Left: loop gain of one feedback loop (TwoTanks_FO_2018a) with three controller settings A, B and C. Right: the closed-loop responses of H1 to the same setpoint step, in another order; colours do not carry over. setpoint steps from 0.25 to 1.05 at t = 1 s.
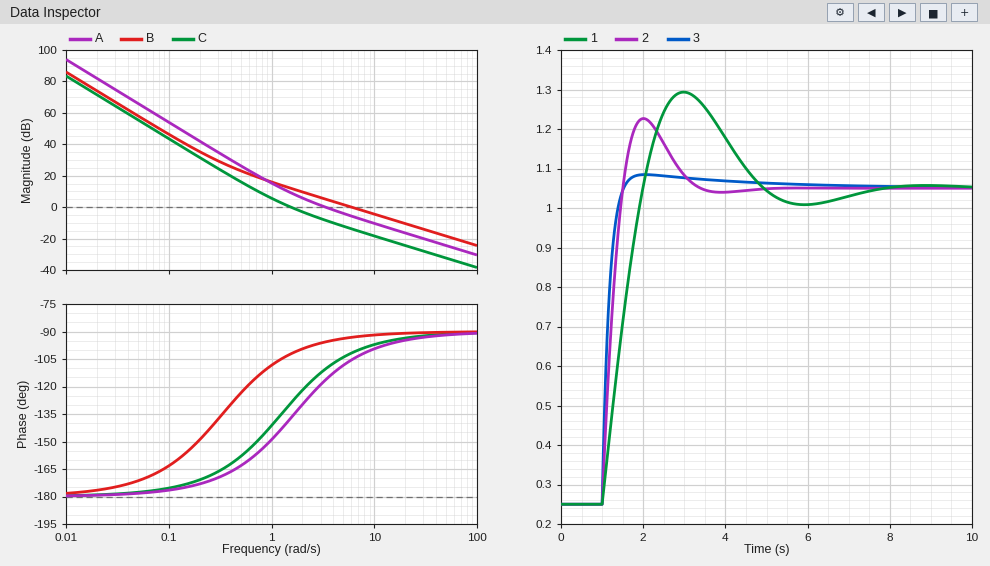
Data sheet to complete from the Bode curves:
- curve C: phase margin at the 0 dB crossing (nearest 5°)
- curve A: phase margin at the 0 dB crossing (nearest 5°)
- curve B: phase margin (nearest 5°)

50°
65°
85°
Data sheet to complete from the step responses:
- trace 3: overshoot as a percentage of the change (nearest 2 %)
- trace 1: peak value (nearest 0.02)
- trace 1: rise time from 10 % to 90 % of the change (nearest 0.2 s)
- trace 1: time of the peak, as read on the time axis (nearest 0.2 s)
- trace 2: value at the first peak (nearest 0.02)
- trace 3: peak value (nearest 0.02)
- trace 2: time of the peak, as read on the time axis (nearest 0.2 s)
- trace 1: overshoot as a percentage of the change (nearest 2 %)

4 %
1.30
0.8 s
3.0 s
1.22
1.08
2.0 s
30 %
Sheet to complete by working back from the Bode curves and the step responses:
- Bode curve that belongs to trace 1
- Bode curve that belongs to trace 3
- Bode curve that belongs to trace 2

C
B
A
